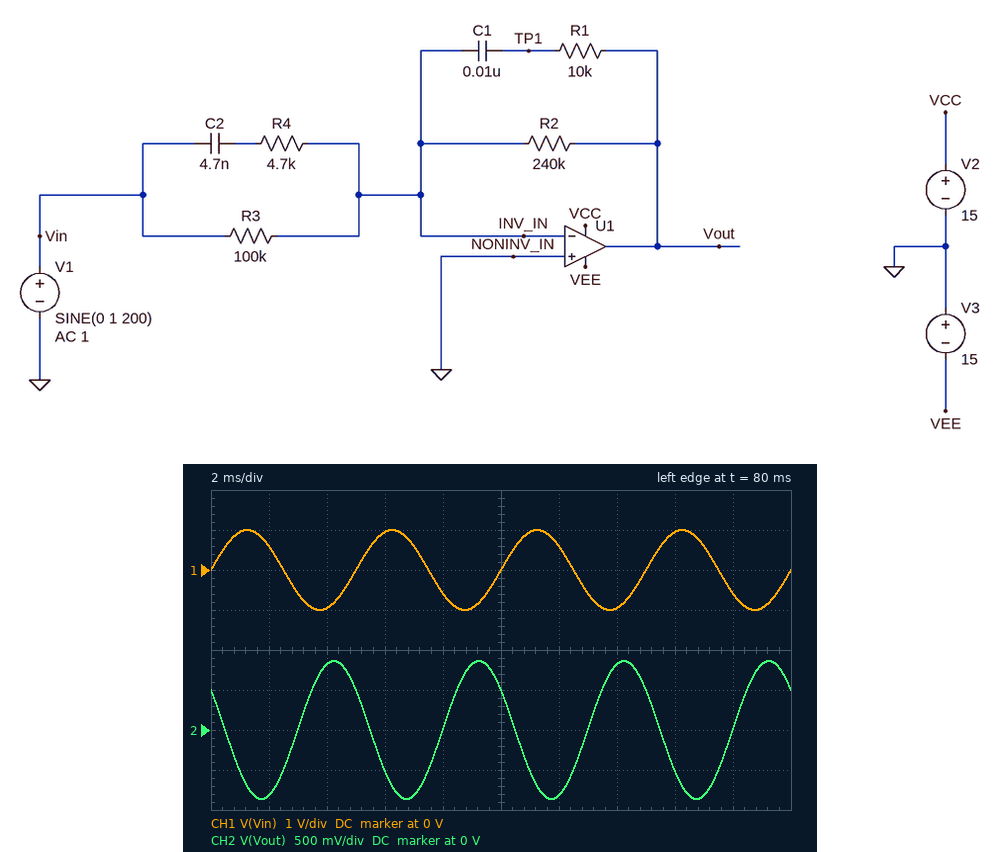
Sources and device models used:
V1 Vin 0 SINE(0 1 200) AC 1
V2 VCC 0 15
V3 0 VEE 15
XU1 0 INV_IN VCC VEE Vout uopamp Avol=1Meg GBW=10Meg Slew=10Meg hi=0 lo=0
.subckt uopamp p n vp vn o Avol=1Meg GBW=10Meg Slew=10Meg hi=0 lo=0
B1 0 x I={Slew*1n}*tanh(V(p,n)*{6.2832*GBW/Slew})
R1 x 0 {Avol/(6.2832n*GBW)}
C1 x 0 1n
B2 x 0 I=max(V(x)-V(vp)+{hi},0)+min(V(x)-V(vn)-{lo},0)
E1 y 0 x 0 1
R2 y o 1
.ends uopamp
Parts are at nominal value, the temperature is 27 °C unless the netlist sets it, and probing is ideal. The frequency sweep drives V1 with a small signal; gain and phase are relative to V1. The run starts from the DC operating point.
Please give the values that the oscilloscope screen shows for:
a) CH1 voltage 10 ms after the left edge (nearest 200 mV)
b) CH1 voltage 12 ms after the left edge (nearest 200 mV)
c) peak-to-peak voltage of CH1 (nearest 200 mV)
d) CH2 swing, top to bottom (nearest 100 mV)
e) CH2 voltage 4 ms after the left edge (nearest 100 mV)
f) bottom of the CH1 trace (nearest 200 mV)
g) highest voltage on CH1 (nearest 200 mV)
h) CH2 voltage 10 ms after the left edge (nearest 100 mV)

0 V
600 mV
2.0 V
1.7 V
800 mV
-1.0 V
1.0 V
500 mV
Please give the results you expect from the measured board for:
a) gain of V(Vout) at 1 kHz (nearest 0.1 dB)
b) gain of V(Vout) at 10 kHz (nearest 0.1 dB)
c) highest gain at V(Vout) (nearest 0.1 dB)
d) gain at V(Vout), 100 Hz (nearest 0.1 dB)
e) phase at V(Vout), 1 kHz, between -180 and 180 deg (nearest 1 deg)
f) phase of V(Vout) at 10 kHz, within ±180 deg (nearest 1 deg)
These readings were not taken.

-4.7 dB
4.9 dB
7.6 dB
2.6 dB
-170 deg
-155 deg
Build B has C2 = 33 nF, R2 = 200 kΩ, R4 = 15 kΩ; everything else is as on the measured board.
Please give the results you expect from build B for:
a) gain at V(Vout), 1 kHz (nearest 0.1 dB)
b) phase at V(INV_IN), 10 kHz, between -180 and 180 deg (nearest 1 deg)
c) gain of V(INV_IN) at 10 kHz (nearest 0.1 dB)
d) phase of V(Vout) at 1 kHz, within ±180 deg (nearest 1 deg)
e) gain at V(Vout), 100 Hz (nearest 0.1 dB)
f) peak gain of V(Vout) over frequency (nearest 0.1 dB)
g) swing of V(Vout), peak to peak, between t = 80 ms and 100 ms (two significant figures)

2.3 dB
83 deg
-62.6 dB
142 deg
9.5 dB
9.7 dB
5.9 V
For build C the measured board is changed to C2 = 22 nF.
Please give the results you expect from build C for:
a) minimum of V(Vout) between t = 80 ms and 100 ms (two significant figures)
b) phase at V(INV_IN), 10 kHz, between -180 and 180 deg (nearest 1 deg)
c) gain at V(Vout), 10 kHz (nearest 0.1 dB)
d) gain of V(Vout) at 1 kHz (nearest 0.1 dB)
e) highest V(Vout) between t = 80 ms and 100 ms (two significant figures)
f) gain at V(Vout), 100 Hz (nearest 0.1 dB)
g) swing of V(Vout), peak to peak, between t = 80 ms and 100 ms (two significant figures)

-2.2 V
89 deg
6.6 dB
6.8 dB
2.2 V
7.1 dB
4.5 V
